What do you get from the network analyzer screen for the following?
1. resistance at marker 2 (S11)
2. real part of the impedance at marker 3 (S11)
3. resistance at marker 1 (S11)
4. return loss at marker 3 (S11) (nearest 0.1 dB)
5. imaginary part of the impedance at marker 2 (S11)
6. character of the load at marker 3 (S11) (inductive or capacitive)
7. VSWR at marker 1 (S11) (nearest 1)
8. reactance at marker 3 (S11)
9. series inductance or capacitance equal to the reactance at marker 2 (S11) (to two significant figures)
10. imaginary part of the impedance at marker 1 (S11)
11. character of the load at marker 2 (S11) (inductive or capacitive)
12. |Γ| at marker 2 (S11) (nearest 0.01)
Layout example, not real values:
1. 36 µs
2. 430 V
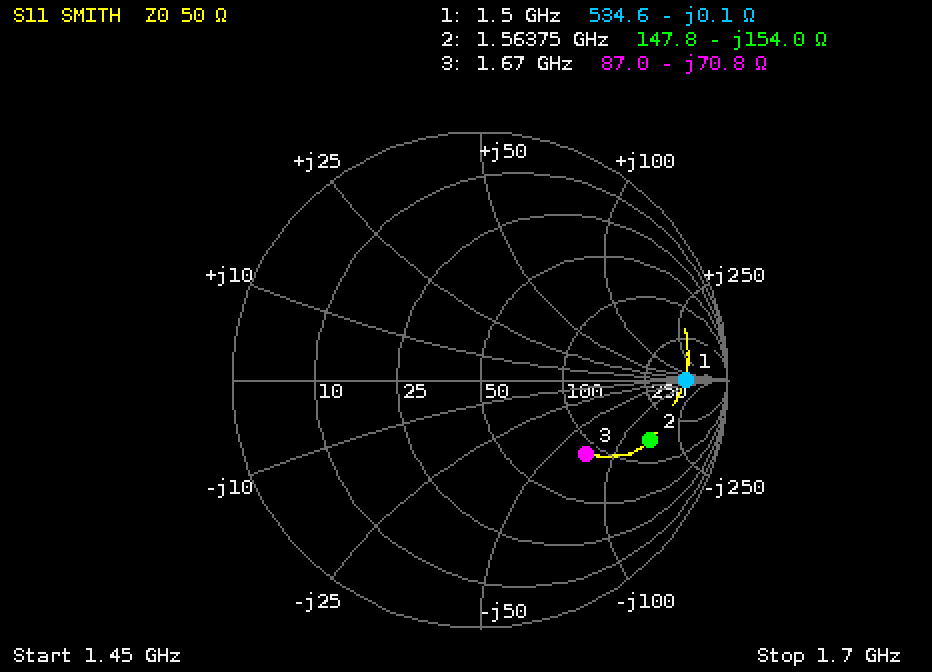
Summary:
1. 147.8 Ω
2. 87.0 Ω
3. 534.6 Ω
4. 5.7 dB
5. -154.0 Ω
6. capacitive
7. 11
8. -70.8 Ω
9. 660 fF
10. -0.1 Ω
11. capacitive
12. 0.73
